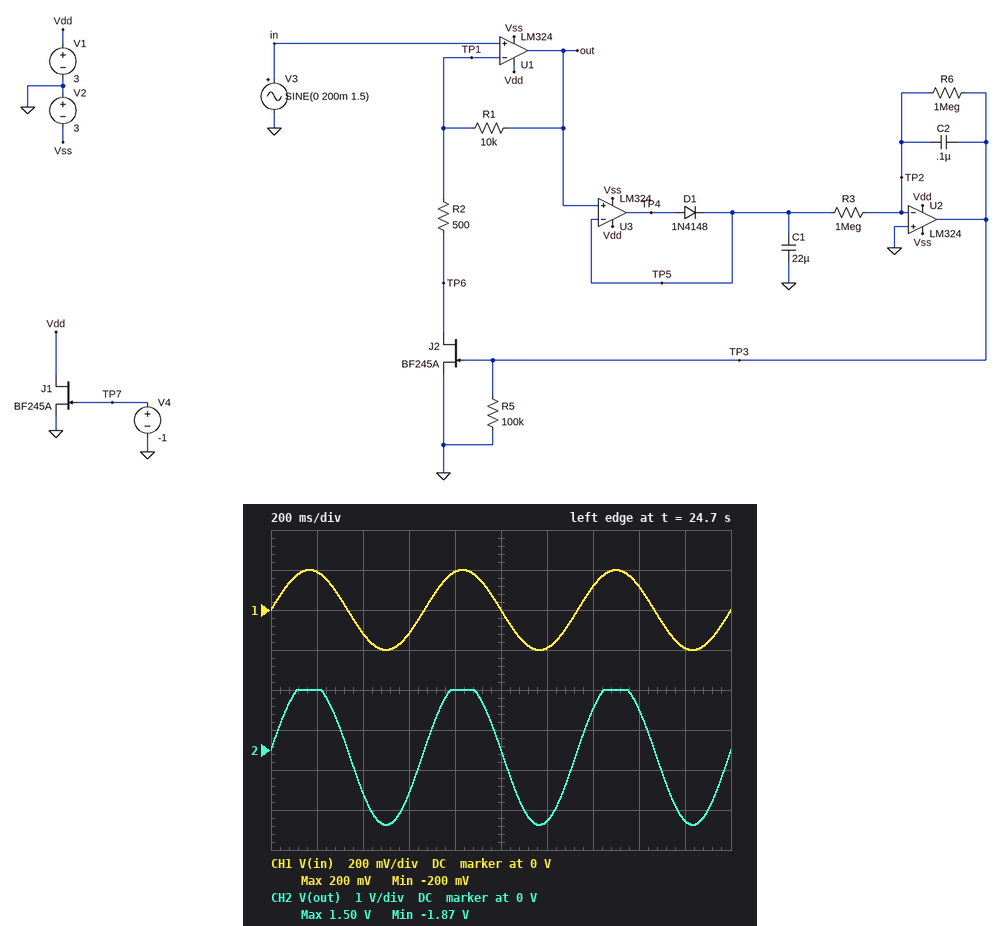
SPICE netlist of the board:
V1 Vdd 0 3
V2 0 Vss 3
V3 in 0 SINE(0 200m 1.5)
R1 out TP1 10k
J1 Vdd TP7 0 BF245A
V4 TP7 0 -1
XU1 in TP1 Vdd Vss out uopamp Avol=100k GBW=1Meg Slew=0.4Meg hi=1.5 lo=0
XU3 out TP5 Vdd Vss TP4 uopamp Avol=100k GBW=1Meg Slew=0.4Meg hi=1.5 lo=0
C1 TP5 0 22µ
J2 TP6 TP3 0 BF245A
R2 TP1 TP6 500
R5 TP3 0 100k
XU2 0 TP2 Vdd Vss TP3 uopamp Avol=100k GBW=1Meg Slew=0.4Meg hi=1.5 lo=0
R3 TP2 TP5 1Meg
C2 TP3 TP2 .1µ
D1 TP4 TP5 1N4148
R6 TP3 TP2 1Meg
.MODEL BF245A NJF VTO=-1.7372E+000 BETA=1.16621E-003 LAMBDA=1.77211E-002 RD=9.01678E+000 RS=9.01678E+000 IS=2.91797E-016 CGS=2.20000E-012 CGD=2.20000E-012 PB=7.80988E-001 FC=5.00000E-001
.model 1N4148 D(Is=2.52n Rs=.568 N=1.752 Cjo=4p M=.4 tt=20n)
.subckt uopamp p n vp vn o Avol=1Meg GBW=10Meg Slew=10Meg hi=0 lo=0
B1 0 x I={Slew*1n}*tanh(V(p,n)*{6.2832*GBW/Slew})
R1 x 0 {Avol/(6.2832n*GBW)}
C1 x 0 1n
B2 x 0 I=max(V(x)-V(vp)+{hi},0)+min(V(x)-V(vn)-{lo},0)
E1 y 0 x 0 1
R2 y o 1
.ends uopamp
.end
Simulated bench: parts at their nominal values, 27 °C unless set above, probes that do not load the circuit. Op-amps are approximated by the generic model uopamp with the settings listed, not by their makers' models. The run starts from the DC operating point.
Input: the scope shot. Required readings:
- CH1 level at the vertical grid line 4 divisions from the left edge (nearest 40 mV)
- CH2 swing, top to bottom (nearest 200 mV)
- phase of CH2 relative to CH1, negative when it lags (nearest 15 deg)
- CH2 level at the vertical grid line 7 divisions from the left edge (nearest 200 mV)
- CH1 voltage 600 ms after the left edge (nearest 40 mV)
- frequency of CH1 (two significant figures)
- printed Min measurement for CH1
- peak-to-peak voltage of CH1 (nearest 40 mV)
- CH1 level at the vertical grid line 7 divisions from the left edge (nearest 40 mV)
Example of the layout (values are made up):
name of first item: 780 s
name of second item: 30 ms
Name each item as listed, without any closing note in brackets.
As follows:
CH1 level at the vertical grid line 4 divisions from the left edge: 200 mV
CH2 swing, top to bottom: 3.4 V
phase of CH2 relative to CH1, negative when it lags: 0 deg
CH2 level at the vertical grid line 7 divisions from the left edge: 1.0 V
CH1 voltage 600 ms after the left edge: -120 mV
frequency of CH1: 1.5 Hz
printed Min measurement for CH1: -200 mV
peak-to-peak voltage of CH1: 400 mV
CH1 level at the vertical grid line 7 divisions from the left edge: 120 mV
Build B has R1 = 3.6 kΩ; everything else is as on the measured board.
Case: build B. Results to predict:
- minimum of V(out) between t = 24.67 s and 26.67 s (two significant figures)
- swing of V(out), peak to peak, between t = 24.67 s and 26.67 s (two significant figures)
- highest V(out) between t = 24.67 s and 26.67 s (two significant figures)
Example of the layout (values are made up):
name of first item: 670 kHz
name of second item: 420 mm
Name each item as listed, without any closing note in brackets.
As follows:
minimum of V(out) between t = 24.67 s and 26.67 s: -930 mV
swing of V(out), peak to peak, between t = 24.67 s and 26.67 s: 1.8 V
highest V(out) between t = 24.67 s and 26.67 s: 890 mV
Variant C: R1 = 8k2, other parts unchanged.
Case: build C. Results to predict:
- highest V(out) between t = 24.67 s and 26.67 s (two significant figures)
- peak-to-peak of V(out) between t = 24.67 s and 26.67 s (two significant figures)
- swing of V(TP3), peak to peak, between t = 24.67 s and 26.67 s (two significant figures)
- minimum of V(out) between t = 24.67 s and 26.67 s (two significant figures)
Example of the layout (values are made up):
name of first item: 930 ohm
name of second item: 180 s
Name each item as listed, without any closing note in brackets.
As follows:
highest V(out) between t = 24.67 s and 26.67 s: 1.4 V
peak-to-peak of V(out) between t = 24.67 s and 26.67 s: 3.0 V
swing of V(TP3), peak to peak, between t = 24.67 s and 26.67 s: 17 mV
minimum of V(out) between t = 24.67 s and 26.67 s: -1.6 V
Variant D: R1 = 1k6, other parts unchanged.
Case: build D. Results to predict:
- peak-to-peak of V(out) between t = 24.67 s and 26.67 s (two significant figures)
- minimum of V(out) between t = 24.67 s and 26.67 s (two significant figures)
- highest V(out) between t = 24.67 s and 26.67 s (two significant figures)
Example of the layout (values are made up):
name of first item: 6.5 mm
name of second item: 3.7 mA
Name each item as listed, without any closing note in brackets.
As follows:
peak-to-peak of V(out) between t = 24.67 s and 26.67 s: 1.1 V
minimum of V(out) between t = 24.67 s and 26.67 s: -570 mV
highest V(out) between t = 24.67 s and 26.67 s: 560 mV
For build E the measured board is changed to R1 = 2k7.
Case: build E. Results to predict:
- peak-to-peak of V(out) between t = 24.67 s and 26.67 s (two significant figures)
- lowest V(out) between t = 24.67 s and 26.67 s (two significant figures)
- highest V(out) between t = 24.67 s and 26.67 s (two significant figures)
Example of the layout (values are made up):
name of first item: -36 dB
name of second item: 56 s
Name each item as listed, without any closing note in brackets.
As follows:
peak-to-peak of V(out) between t = 24.67 s and 26.67 s: 1.5 V
lowest V(out) between t = 24.67 s and 26.67 s: -780 mV
highest V(out) between t = 24.67 s and 26.67 s: 760 mV
